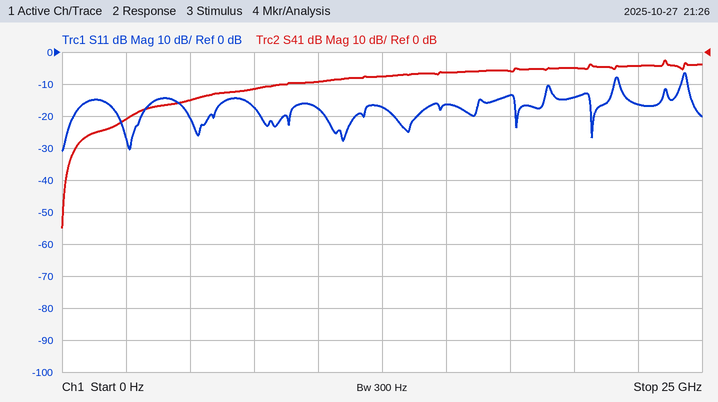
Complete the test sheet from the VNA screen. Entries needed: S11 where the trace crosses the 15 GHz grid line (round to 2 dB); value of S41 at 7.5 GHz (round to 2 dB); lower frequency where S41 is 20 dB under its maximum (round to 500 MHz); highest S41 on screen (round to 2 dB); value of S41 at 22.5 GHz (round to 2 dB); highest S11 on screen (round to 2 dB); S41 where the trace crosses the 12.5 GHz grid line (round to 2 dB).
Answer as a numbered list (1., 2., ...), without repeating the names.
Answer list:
1. -16 dB
2. -12 dB
3. 2.0 GHz
4. -2 dB
5. -4 dB
6. -6 dB
7. -8 dB
